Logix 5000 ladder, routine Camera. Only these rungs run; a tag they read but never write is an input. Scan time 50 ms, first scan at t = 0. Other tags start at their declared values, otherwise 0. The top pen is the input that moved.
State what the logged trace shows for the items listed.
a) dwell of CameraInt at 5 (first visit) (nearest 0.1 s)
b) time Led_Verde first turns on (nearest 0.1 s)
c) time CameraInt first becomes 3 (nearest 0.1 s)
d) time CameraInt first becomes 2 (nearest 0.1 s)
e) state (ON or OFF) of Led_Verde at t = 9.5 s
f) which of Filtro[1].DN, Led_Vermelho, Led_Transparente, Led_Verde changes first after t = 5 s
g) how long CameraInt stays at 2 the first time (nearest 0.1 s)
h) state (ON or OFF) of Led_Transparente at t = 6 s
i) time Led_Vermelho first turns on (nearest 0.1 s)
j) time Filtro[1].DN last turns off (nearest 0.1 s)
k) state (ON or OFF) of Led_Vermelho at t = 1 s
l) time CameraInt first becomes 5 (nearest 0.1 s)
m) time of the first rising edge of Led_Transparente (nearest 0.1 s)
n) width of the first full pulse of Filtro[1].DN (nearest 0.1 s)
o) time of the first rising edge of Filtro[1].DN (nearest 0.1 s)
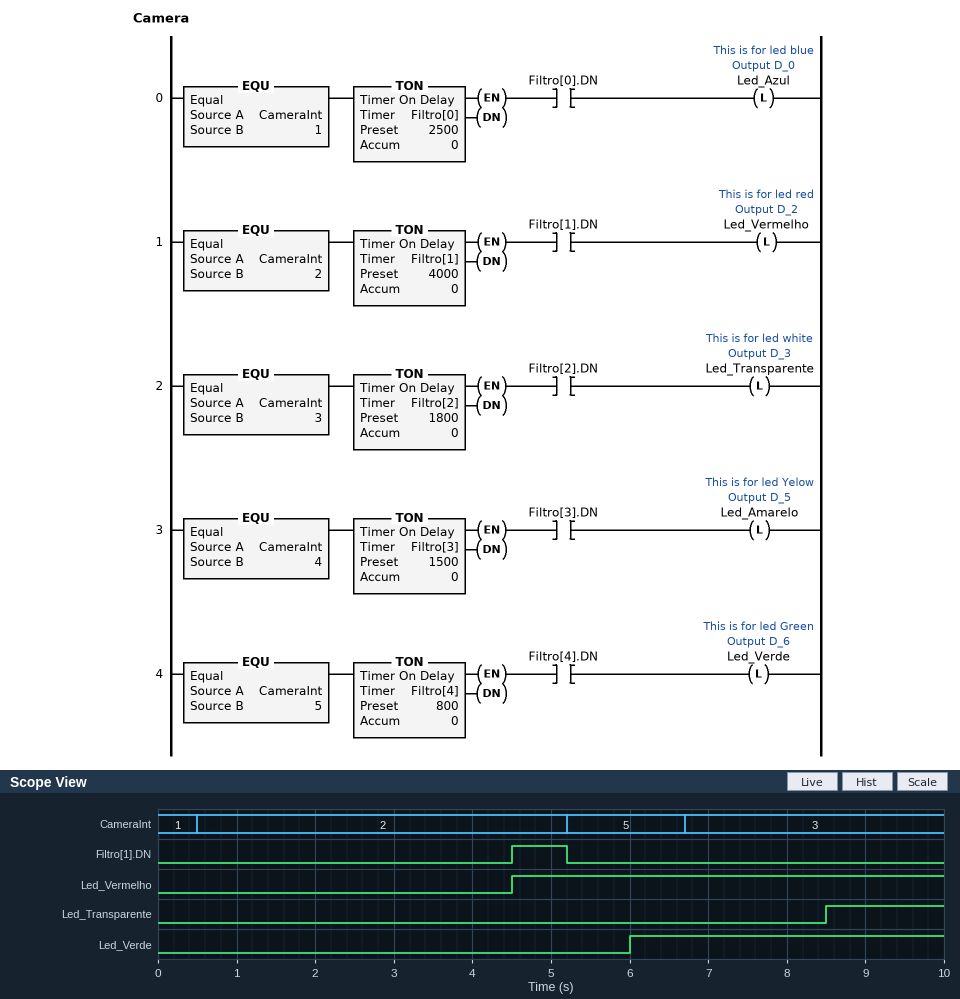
1.5 s
6.0 s
6.7 s
0.5 s
ON
Filtro[1].DN
4.7 s
OFF
4.5 s
5.2 s
OFF
5.2 s
8.5 s
0.7 s
4.5 s
